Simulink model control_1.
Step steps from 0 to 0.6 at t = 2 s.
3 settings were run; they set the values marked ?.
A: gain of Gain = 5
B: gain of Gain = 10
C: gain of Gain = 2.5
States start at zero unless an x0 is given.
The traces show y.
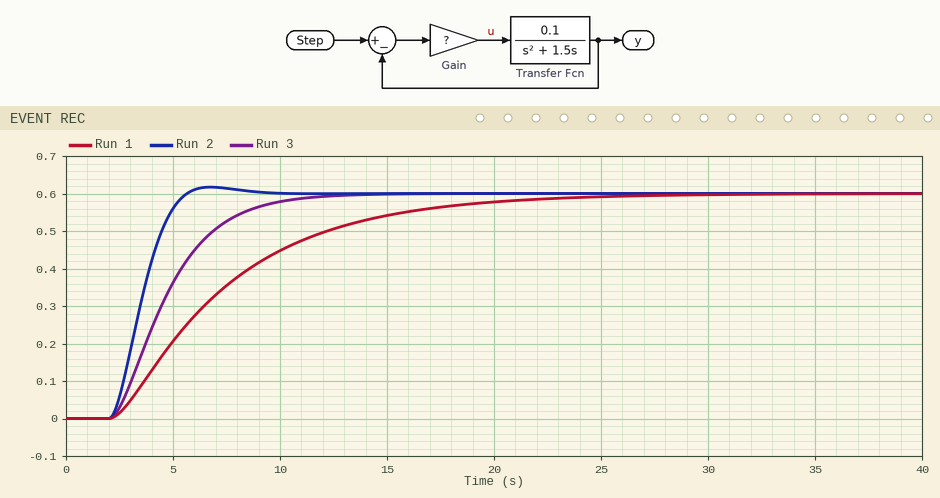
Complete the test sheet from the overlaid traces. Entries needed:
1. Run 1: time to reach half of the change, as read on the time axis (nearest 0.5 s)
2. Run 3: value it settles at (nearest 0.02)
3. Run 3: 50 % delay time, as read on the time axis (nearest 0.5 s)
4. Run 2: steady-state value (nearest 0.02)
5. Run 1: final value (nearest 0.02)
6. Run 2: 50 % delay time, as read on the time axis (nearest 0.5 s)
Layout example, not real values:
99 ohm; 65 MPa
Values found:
6.5 s; 0.60; 4.5 s; 0.60; 0.60; 3.5 s
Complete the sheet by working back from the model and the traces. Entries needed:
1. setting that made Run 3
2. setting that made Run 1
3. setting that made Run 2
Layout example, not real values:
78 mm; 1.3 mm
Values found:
A; C; B
